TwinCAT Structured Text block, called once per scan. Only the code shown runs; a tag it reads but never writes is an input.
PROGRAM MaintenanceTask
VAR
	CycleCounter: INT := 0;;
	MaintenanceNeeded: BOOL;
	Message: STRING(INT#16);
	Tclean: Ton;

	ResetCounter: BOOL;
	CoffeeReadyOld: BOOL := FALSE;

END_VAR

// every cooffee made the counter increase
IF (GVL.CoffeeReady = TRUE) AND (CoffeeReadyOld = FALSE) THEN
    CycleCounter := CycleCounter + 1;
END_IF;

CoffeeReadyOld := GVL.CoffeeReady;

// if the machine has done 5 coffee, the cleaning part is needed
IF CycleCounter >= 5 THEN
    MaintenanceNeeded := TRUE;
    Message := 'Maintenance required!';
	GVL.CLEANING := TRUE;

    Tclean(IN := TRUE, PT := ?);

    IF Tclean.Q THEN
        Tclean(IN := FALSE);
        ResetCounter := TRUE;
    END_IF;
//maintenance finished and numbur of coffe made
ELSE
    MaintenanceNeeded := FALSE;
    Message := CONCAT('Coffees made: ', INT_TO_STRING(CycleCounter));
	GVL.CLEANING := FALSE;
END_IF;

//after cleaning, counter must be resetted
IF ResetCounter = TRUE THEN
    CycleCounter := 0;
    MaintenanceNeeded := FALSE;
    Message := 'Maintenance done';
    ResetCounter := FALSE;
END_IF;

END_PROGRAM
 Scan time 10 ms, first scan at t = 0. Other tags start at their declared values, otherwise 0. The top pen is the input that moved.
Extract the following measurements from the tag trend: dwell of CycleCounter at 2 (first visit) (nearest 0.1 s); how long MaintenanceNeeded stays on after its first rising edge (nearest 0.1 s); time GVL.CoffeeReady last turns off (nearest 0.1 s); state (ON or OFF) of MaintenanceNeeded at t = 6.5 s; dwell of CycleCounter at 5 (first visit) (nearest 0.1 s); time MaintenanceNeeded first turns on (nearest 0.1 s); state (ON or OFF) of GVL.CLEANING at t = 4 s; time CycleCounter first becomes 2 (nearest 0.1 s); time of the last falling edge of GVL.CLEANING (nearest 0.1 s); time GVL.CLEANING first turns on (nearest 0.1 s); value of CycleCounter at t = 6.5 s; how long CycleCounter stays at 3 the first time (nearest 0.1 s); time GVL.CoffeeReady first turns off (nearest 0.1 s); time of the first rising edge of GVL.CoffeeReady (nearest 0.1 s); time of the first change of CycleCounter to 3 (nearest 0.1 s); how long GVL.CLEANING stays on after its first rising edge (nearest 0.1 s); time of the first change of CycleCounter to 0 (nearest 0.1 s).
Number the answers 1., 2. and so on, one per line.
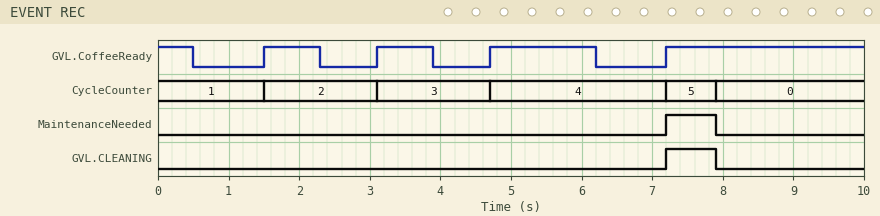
1. 1.6 s
2. 0.7 s
3. 6.2 s
4. OFF
5. 0.7 s
6. 7.2 s
7. OFF
8. 1.5 s
9. 7.9 s
10. 7.2 s
11. 4
12. 1.6 s
13. 0.5 s
14. 1.5 s
15. 3.1 s
16. 0.7 s
17. 7.9 s
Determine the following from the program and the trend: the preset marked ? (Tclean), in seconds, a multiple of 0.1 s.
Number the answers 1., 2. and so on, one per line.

1. 0.7 s
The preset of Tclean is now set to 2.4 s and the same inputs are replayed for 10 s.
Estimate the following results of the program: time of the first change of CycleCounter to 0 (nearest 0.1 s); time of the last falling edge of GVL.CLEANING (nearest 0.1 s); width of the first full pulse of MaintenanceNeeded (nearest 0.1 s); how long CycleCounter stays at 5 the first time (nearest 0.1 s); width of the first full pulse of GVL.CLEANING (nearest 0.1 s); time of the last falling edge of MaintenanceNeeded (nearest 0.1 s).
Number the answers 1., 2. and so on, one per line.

1. 9.6 s
2. 9.6 s
3. 2.4 s
4. 2.4 s
5. 2.4 s
6. 9.6 s
